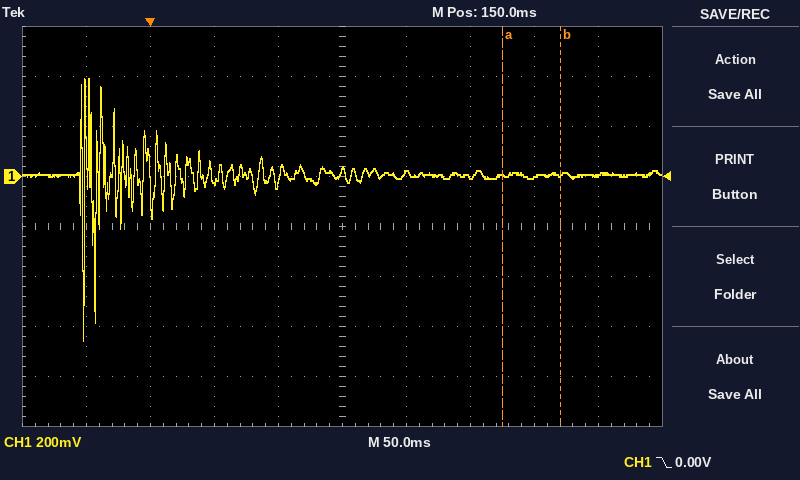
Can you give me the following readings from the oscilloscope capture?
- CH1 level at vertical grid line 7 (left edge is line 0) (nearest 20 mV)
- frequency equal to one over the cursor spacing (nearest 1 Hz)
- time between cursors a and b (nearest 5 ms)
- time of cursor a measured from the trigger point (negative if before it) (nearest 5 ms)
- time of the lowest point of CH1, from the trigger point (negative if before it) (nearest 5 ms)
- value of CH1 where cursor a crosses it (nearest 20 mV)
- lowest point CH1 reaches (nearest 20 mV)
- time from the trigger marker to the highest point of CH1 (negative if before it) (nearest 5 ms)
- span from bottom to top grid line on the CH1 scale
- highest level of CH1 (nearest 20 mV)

0 mV
22 Hz
45 ms
+275 ms
-50 ms
0 mV
-660 mV
-50 ms
1.6 V
400 mV
